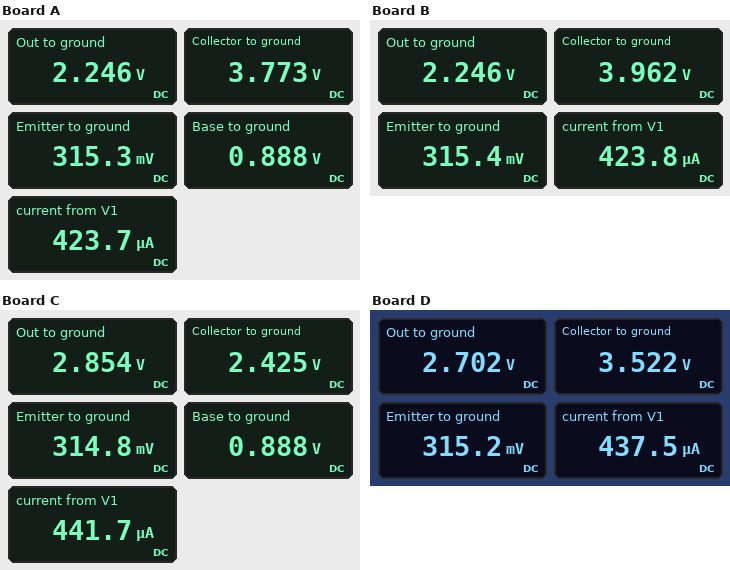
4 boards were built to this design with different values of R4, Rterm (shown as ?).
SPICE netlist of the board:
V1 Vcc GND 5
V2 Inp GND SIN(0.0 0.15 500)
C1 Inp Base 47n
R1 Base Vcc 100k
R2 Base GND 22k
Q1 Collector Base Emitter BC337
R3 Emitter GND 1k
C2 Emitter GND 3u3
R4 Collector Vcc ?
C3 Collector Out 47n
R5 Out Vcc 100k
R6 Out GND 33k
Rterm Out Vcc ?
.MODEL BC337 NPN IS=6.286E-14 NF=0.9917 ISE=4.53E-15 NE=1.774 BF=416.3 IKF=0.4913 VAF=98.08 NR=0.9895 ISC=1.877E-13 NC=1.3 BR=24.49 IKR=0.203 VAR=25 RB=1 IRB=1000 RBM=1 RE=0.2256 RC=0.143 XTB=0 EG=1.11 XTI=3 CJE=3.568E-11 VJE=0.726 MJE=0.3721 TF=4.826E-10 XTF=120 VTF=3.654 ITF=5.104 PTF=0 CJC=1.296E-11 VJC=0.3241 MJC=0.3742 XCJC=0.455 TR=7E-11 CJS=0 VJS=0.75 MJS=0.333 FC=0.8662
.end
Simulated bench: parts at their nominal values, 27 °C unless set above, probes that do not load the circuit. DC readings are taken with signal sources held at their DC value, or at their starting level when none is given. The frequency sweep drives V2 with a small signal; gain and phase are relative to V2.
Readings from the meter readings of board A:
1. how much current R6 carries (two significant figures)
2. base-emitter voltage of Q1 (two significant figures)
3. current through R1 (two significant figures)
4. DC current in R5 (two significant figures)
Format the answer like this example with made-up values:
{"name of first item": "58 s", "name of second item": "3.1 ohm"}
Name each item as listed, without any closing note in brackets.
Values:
{"how much current R6 carries": "68 µA", "base-emitter voltage of Q1": "570 mV", "current through R1": "41 µA", "DC current in R5": "28 µA"}
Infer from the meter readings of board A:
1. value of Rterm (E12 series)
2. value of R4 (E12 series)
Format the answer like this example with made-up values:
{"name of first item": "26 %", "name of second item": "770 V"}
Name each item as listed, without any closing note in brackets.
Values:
{"value of Rterm": "68 kΩ", "value of R4": "3.9 kΩ"}
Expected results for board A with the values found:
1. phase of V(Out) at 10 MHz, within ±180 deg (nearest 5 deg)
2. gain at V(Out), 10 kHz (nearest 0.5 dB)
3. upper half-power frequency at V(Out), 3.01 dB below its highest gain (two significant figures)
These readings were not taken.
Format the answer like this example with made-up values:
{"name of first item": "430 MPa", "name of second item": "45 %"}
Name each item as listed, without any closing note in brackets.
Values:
{"phase of V(Out) at 10 MHz, within ±180 deg": "130 deg", "gain at V(Out), 10 kHz": "31.5 dB", "upper half-power frequency at V(Out), 3.01 dB below its highest gain": "9.1 MHz"}
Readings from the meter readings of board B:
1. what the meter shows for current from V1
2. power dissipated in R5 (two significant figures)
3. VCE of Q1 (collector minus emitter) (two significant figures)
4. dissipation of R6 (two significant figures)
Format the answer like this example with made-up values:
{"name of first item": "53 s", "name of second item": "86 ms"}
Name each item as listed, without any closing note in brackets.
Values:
{"what the meter shows for current from V1": "423.8 µA", "power dissipated in R5": "76 µW", "VCE of Q1 (collector minus emitter)": "3.6 V", "dissipation of R6": "150 µW"}
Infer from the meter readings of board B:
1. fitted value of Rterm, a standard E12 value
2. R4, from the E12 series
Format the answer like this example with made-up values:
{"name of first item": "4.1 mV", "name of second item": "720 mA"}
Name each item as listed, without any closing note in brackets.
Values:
{"fitted value of Rterm, a standard E12 value": "68 kΩ", "R4, from the E12 series": "3.3 kΩ"}
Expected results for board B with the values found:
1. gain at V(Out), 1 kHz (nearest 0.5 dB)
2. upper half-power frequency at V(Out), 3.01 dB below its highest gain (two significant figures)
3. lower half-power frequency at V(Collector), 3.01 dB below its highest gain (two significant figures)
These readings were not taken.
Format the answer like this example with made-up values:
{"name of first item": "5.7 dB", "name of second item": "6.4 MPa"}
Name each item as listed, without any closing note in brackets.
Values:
{"gain at V(Out), 1 kHz": "28.5 dB", "upper half-power frequency at V(Out), 3.01 dB below its highest gain": "11 MHz", "lower half-power frequency at V(Collector), 3.01 dB below its highest gain": "770 Hz"}
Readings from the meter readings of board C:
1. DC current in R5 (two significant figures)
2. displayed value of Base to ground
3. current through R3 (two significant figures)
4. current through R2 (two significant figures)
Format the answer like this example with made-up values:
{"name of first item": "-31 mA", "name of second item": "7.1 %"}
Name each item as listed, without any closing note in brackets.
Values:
{"DC current in R5": "21 µA", "displayed value of Base to ground": "0.888 V", "current through R3": "310 µA", "current through R2": "40 µA"}
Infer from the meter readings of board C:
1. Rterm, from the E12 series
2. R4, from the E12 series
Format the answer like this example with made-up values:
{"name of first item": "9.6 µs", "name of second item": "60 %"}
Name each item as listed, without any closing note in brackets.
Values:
{"Rterm, from the E12 series": "33 kΩ", "R4, from the E12 series": "8.2 kΩ"}
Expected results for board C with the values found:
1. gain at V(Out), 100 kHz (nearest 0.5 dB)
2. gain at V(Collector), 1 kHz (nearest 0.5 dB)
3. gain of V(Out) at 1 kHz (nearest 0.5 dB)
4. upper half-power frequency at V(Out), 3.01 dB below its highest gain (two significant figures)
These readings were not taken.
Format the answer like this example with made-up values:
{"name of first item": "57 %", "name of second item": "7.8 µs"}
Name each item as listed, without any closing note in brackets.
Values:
{"gain at V(Out), 100 kHz": "36.0 dB", "gain at V(Collector), 1 kHz": "34.0 dB", "gain of V(Out) at 1 kHz": "33.5 dB", "upper half-power frequency at V(Out), 3.01 dB below its highest gain": "4.6 MHz"}
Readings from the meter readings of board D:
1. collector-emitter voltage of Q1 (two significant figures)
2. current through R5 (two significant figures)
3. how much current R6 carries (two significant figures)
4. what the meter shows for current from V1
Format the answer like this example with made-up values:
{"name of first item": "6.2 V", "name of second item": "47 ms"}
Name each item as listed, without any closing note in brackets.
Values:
{"collector-emitter voltage of Q1": "3.2 V", "current through R5": "23 µA", "how much current R6 carries": "82 µA", "what the meter shows for current from V1": "437.5 µA"}
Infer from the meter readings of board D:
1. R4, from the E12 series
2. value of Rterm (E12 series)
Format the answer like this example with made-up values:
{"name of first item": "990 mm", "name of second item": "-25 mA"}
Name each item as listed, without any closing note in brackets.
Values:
{"R4, from the E12 series": "4.7 kΩ", "value of Rterm": "39 kΩ"}
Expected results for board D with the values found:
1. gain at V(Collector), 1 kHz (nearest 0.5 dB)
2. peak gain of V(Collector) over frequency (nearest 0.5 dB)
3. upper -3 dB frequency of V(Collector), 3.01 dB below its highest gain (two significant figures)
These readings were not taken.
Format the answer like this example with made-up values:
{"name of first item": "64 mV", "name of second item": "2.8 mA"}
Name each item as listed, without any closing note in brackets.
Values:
{"gain at V(Collector), 1 kHz": "30.5 dB", "peak gain of V(Collector) over frequency": "32.5 dB", "upper -3 dB frequency of V(Collector), 3.01 dB below its highest gain": "7.9 MHz"}
